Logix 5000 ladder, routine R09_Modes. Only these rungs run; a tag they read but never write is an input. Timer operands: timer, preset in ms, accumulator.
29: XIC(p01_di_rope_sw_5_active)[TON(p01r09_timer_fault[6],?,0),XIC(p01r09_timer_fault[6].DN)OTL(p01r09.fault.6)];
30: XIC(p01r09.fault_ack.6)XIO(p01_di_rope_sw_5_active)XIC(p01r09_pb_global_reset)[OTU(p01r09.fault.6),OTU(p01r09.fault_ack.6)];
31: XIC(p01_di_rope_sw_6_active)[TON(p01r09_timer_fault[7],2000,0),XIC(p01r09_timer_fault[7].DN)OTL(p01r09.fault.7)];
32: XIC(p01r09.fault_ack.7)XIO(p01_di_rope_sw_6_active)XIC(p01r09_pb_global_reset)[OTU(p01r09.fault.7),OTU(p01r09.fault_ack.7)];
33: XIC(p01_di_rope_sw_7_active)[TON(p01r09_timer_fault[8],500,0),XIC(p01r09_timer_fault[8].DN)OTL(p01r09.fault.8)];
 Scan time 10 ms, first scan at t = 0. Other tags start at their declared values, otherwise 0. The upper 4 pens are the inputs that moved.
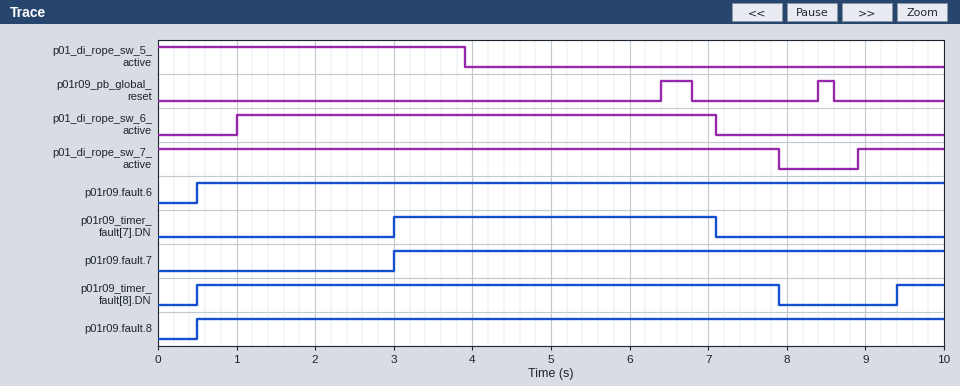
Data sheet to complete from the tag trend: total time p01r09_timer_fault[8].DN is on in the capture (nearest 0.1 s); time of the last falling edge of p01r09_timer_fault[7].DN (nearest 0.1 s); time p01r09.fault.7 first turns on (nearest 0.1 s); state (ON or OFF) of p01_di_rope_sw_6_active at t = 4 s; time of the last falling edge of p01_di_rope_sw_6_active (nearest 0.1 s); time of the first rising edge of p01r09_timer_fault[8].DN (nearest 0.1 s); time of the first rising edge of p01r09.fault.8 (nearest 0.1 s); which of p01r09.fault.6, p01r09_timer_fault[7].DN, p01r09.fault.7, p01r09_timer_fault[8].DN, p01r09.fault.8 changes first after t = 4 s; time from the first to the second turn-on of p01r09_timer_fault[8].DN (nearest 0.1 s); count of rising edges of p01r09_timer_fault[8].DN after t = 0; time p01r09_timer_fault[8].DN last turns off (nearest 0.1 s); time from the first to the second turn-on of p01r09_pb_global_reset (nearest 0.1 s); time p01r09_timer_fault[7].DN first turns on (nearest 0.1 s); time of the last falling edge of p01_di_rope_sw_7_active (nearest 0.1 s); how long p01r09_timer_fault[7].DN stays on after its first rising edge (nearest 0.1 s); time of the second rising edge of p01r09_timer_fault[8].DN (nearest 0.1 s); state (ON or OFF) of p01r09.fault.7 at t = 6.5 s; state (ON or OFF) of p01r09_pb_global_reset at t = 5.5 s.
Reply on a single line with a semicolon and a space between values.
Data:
8.0 s; 7.1 s; 3.0 s; ON; 7.1 s; 0.5 s; 0.5 s; p01r09_timer_fault[7].DN; 8.9 s; 2; 7.9 s; 2.0 s; 3.0 s; 7.9 s; 4.1 s; 9.4 s; ON; OFF
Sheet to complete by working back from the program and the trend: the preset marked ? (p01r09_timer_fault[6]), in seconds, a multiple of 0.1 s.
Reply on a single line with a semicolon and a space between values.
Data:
0.5 s
